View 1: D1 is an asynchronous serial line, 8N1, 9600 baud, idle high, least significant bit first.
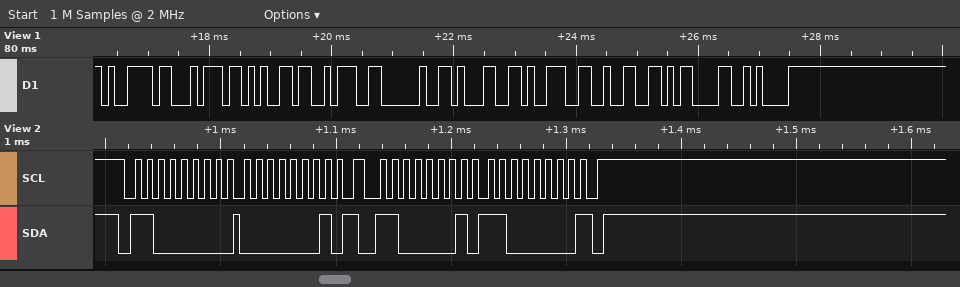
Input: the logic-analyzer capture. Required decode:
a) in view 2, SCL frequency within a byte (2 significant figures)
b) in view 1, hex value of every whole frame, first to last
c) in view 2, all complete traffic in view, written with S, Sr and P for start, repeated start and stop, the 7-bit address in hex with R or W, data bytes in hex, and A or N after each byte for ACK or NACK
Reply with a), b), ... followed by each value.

a) 100 kHz
b) 79 74 65 3A 20 31 39 32 0D 0A
c) S 60W A 01 A Sr 60R A C0 N P
